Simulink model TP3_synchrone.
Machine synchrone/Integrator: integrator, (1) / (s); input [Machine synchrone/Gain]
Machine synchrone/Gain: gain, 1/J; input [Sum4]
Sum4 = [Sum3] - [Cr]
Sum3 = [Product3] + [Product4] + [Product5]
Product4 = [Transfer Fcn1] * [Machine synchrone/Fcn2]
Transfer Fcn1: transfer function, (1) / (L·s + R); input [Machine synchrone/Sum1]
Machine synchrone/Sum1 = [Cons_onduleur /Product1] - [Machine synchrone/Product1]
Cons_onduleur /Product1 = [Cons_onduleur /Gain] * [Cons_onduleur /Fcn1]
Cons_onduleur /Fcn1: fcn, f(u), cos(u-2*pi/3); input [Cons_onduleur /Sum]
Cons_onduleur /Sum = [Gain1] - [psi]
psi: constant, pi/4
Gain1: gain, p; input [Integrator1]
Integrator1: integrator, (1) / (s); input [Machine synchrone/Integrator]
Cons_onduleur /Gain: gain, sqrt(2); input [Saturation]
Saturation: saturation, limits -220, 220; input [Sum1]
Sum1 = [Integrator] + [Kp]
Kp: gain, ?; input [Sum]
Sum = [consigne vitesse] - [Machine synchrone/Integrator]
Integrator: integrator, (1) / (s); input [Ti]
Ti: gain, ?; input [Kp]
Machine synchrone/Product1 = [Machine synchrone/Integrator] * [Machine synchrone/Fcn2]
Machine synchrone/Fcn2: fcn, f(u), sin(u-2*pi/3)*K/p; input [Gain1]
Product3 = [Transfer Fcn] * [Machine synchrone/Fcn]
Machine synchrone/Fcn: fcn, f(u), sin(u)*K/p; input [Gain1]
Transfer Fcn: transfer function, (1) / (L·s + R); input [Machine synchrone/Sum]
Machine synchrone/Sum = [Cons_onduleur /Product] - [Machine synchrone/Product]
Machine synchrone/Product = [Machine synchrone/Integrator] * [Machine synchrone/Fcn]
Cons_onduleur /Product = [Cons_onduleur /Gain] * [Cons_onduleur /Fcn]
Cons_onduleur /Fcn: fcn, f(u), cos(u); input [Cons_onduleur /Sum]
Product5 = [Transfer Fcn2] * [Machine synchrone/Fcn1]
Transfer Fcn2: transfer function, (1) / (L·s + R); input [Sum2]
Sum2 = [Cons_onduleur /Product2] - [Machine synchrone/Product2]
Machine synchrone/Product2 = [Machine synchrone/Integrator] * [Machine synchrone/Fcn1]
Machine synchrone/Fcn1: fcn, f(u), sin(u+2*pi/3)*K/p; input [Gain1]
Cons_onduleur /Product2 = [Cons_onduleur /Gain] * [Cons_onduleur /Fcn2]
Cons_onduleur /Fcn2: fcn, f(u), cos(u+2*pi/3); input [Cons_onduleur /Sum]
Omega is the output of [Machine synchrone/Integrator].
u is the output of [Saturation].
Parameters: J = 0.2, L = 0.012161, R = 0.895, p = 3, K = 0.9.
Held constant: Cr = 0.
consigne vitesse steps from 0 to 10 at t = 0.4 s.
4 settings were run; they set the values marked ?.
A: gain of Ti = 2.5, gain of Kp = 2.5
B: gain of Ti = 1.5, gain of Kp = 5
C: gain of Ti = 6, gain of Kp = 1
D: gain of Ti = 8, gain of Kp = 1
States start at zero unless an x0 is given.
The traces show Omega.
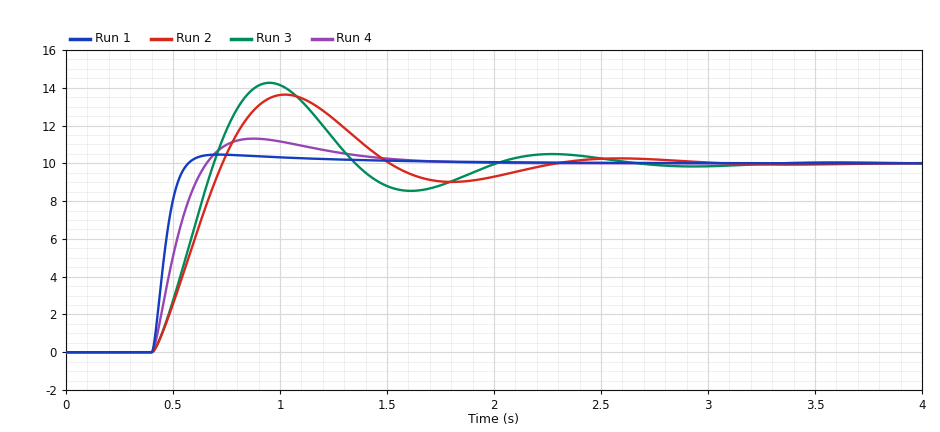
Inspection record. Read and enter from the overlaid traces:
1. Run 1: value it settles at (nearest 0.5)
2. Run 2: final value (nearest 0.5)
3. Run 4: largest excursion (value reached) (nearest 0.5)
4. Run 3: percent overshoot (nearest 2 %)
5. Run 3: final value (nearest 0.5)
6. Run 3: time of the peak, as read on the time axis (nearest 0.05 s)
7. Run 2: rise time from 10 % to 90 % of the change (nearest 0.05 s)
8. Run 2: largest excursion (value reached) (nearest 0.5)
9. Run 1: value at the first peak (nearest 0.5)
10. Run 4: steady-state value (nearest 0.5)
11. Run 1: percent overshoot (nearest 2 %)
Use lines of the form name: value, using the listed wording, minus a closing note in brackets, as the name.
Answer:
Run 1: value it settles at: 10.0
Run 2: final value: 10.0
Run 4: largest excursion (value reached): 11.5
Run 3: percent overshoot: 42 %
Run 3: final value: 10.0
Run 3: time of the peak, as read on the time axis: 0.95 s
Run 2: rise time from 10 % to 90 % of the change: 0.25 s
Run 2: largest excursion (value reached): 13.5
Run 1: value at the first peak: 10.5
Run 4: steady-state value: 10.0
Run 1: percent overshoot: 4 %
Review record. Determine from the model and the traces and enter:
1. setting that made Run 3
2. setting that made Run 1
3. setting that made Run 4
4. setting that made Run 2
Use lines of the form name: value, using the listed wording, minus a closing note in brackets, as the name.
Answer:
setting that made Run 3: D
setting that made Run 1: B
setting that made Run 4: A
setting that made Run 2: C
